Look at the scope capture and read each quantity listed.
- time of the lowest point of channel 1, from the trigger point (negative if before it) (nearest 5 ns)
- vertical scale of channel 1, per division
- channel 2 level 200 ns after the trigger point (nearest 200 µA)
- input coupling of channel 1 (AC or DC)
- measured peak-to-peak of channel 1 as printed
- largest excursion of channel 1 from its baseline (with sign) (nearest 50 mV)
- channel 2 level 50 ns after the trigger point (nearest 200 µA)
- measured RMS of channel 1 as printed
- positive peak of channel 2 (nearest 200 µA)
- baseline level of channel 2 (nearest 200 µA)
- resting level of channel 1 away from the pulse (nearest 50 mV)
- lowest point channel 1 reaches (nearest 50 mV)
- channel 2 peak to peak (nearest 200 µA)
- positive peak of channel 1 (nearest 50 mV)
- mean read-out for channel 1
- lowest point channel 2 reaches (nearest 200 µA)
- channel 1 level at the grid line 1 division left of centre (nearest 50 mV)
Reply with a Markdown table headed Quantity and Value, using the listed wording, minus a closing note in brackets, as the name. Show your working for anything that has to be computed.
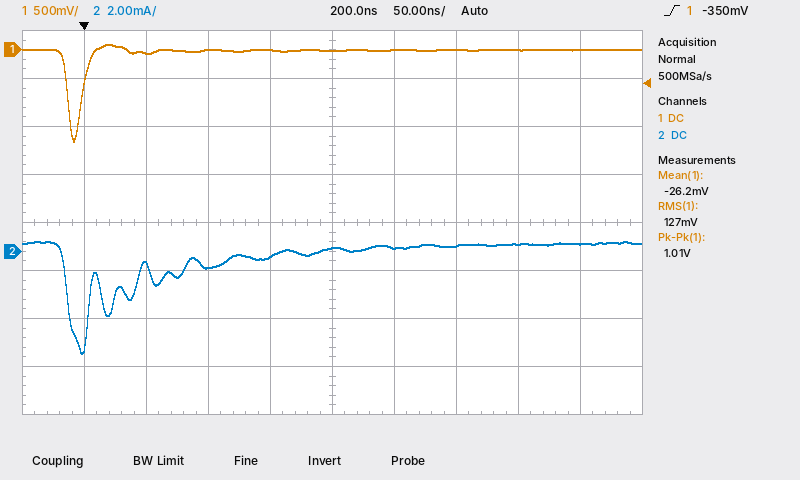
| Quantity | Value |
|---|---|
| time of the lowest point of channel 1, from the trigger point (negative if before it) | -10 ns |
| vertical scale of channel 1, per division | 500 mV |
| channel 2 level 200 ns after the trigger point | 200 µA |
| input coupling of channel 1 | DC |
| measured peak-to-peak of channel 1 as printed | 1.01 V |
| largest excursion of channel 1 from its baseline (with sign) | -950 mV − (0 mV) = -950 mV |
| channel 2 level 50 ns after the trigger point | -600 µA |
| measured RMS of channel 1 as printed | 127 mV |
| positive peak of channel 2 | 400 µA |
| baseline level of channel 2 | 200 µA |
| resting level of channel 1 away from the pulse | 0 mV |
| lowest point channel 1 reaches | -950 mV |
| channel 2 peak to peak | 400 µA − (-4.2 mA) = 4.6 mA |
| positive peak of channel 1 | 50 mV |
| mean read-out for channel 1 | -26.2 mV |
| lowest point channel 2 reaches | -4.2 mA |
| channel 1 level at the grid line 1 division left of centre | 0 mV |
